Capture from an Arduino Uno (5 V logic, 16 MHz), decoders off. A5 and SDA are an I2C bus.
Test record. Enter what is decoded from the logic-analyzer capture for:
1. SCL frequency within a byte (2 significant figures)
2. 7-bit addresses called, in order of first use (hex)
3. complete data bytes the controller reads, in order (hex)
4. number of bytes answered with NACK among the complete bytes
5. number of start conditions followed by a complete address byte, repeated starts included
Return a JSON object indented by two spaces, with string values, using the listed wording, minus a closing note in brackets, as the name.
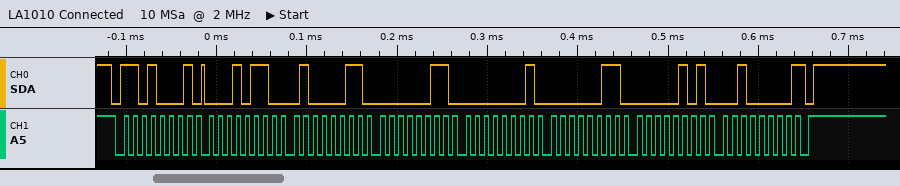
{
  "SCL frequency within a byte": "100 kHz",
  "7-bit addresses called, in order of first use": "0x68",
  "complete data bytes the controller reads, in order": "16 43 03 01 03 05 20",
  "number of bytes answered with NACK among the complete bytes": "1",
  "number of start conditions followed by a complete address byte, repeated starts included": "1"
}
